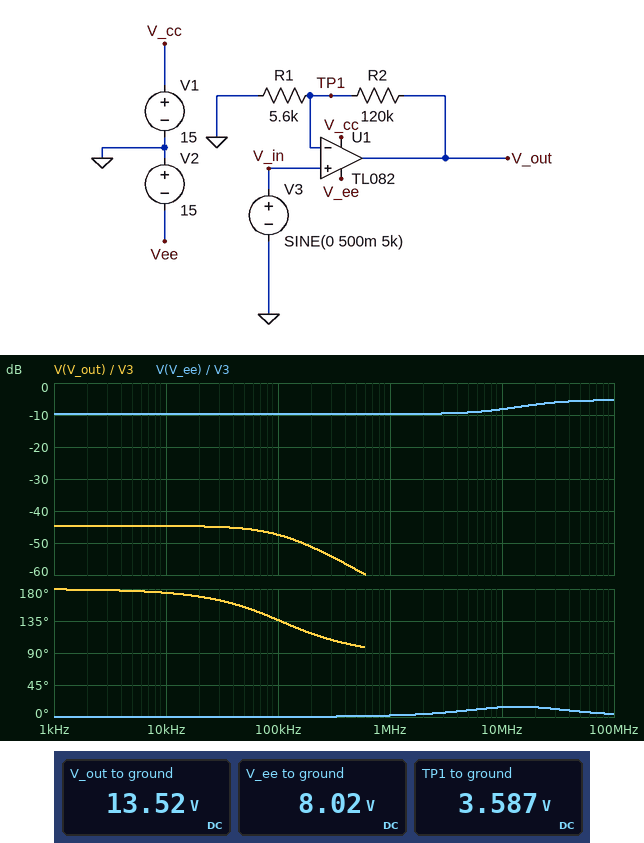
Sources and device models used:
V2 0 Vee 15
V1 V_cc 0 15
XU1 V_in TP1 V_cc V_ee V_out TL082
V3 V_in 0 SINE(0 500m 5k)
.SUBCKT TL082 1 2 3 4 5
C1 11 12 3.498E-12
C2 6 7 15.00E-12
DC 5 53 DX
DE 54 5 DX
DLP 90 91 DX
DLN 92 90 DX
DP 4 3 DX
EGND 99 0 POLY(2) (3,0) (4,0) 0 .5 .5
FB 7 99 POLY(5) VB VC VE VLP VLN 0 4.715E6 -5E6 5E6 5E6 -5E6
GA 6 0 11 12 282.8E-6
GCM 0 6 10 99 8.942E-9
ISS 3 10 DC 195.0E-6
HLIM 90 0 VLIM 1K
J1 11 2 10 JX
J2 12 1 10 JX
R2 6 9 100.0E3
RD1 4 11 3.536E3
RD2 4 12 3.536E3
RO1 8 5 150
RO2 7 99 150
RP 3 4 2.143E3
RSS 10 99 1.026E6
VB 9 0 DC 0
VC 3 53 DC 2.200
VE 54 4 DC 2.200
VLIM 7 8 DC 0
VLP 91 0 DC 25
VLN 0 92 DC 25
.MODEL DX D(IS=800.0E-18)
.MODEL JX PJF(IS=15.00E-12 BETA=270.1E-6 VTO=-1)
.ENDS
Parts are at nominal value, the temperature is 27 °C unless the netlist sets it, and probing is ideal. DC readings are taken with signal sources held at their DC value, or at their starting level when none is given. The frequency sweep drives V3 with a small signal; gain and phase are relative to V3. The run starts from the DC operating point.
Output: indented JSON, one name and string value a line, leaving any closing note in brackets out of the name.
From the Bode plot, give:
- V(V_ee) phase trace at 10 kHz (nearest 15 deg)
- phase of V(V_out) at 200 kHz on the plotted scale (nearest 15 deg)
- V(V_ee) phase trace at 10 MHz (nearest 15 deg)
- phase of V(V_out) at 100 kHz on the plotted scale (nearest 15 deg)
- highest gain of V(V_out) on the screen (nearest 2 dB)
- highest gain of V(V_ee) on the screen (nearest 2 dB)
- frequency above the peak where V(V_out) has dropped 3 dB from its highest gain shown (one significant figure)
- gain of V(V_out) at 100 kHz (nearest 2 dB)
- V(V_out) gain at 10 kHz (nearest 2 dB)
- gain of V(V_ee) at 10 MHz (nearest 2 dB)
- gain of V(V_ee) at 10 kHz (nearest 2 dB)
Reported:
{
  "V(V_ee) phase trace at 10 kHz": "0 deg",
  "phase of V(V_out) at 200 kHz on the plotted scale": "120 deg",
  "V(V_ee) phase trace at 10 MHz": "15 deg",
  "phase of V(V_out) at 100 kHz on the plotted scale": "135 deg",
  "highest gain of V(V_out) on the screen": "-44 dB",
  "highest gain of V(V_ee) on the screen": "-6 dB",
  "frequency above the peak where V(V_out) has dropped 3 dB from its highest gain shown": "100 kHz",
  "gain of V(V_out) at 100 kHz": "-48 dB",
  "V(V_out) gain at 10 kHz": "-44 dB",
  "gain of V(V_ee) at 10 MHz": "-8 dB",
  "gain of V(V_ee) at 10 kHz": "-10 dB"
}
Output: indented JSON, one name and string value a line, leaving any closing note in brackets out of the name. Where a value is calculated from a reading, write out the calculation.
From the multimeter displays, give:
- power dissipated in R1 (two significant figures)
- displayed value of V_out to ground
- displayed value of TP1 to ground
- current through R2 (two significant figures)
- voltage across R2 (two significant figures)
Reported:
{
  "power dissipated in R1": "(3.587 V)^2 / 5.6 kΩ = 2.3 mW",
  "displayed value of V_out to ground": "13.52 V",
  "displayed value of TP1 to ground": "3.587 V",
  "current through R2": "(13.52 V - 3.587 V) / 120 kΩ = 83 µA",
  "voltage across R2": "13.52 V - 3.587 V = 9.9 V"
}
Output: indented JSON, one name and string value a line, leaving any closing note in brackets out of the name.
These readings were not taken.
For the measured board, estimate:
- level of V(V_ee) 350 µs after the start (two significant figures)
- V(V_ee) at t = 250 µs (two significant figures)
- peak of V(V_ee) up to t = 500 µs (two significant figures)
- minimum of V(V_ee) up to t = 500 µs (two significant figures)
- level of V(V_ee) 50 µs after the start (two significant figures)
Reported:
{
  "level of V(V_ee) 350 µs after the start": "7.9 V",
  "V(V_ee) at t = 250 µs": "8.2 V",
  "peak of V(V_ee) up to t = 500 µs": "8.2 V",
  "minimum of V(V_ee) up to t = 500 µs": "7.9 V",
  "level of V(V_ee) 50 µs after the start": "8.2 V"
}
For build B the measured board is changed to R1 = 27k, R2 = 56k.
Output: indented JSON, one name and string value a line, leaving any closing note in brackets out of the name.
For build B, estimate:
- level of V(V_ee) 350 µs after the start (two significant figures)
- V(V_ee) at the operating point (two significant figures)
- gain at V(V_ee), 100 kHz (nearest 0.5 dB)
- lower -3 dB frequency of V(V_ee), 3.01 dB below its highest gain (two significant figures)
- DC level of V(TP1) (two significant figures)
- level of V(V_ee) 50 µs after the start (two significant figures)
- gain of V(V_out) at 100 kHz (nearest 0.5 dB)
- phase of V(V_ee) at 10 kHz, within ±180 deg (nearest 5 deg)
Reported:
{
  "level of V(V_ee) 350 µs after the start": "8.5 V",
  "V(V_ee) at the operating point": "8.7 V",
  "gain at V(V_ee), 100 kHz": "-9.0 dB",
  "lower -3 dB frequency of V(V_ee), 3.01 dB below its highest gain": "5.1 MHz",
  "DC level of V(TP1)": "6.1 V",
  "level of V(V_ee) 50 µs after the start": "8.9 V",
  "gain of V(V_out) at 100 kHz": "-53.0 dB",
  "phase of V(V_ee) at 10 kHz, within ±180 deg": "0 deg"
}
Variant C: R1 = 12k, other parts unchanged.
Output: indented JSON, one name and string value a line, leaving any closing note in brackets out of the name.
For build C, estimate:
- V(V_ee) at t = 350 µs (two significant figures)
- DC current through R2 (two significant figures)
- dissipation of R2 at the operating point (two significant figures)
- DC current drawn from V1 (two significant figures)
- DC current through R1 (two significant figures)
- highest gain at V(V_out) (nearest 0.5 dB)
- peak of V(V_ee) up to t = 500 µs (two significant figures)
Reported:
{
  "V(V_ee) at t = 350 µs": "8.2 V",
  "DC current through R2": "73 µA",
  "dissipation of R2 at the operating point": "640 µW",
  "DC current drawn from V1": "2.0 mA",
  "DC current through R1": "400 µA",
  "highest gain at V(V_out)": "-48.0 dB",
  "peak of V(V_ee) up to t = 500 µs": "8.5 V"
}
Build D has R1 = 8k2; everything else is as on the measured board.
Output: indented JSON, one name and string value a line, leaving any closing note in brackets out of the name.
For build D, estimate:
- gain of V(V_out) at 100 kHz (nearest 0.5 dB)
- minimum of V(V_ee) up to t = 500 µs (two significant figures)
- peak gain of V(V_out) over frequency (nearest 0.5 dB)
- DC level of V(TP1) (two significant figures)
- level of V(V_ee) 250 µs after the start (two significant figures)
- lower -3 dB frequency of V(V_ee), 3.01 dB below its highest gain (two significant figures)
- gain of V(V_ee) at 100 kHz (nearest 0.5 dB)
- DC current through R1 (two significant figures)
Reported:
{
  "gain of V(V_out) at 100 kHz": "-49.0 dB",
  "minimum of V(V_ee) up to t = 500 µs": "8.0 V",
  "peak gain of V(V_out) over frequency": "-46.5 dB",
  "DC level of V(TP1)": "4.2 V",
  "level of V(V_ee) 250 µs after the start": "8.4 V",
  "lower -3 dB frequency of V(V_ee), 3.01 dB below its highest gain": "7.6 MHz",
  "gain of V(V_ee) at 100 kHz": "-9.5 dB",
  "DC current through R1": "510 µA"
}
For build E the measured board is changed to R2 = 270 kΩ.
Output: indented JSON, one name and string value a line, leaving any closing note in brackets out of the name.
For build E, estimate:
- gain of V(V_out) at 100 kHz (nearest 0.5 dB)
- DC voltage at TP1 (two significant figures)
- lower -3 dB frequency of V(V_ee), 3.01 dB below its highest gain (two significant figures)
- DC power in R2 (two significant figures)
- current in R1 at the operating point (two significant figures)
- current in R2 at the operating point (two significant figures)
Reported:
{
  "gain of V(V_out) at 100 kHz": "-47.0 dB",
  "DC voltage at TP1": "3.5 V",
  "lower -3 dB frequency of V(V_ee), 3.01 dB below its highest gain": "9.4 MHz",
  "DC power in R2": "370 µW",
  "current in R1 at the operating point": "620 µA",
  "current in R2 at the operating point": "37 µA"
}
